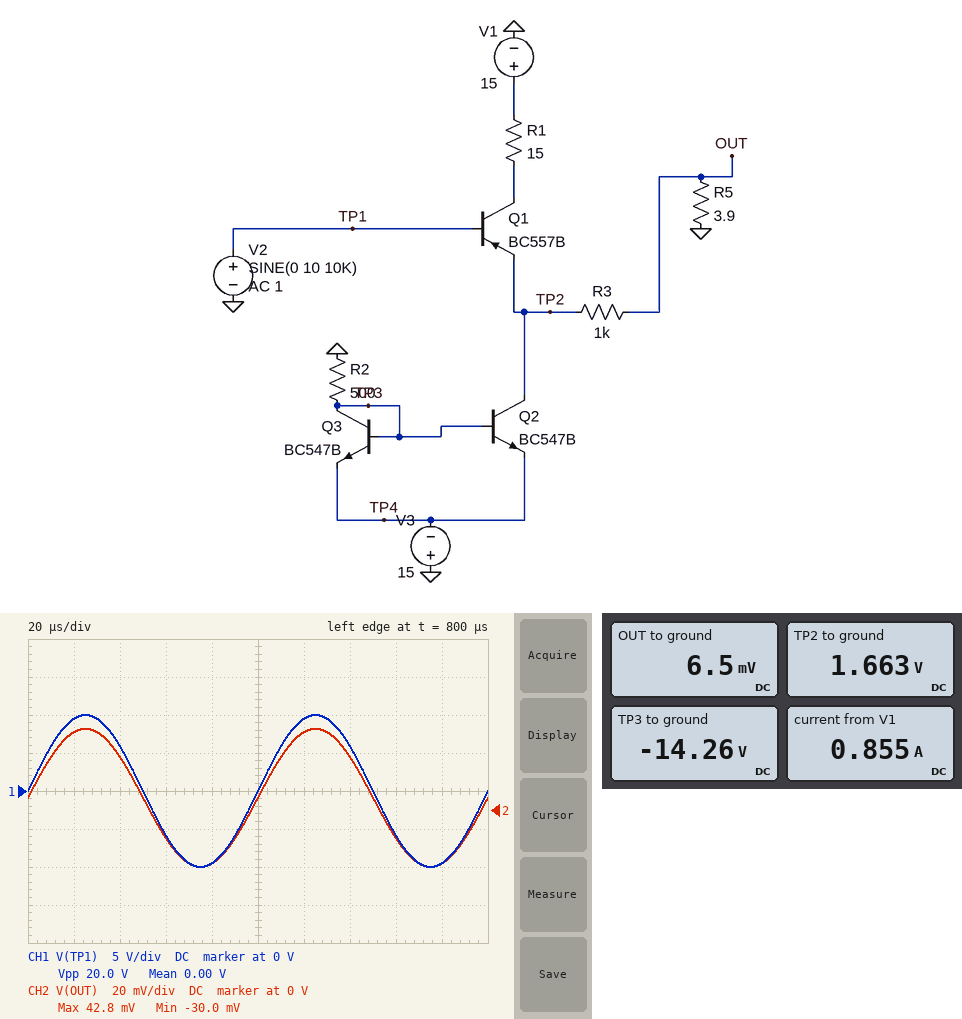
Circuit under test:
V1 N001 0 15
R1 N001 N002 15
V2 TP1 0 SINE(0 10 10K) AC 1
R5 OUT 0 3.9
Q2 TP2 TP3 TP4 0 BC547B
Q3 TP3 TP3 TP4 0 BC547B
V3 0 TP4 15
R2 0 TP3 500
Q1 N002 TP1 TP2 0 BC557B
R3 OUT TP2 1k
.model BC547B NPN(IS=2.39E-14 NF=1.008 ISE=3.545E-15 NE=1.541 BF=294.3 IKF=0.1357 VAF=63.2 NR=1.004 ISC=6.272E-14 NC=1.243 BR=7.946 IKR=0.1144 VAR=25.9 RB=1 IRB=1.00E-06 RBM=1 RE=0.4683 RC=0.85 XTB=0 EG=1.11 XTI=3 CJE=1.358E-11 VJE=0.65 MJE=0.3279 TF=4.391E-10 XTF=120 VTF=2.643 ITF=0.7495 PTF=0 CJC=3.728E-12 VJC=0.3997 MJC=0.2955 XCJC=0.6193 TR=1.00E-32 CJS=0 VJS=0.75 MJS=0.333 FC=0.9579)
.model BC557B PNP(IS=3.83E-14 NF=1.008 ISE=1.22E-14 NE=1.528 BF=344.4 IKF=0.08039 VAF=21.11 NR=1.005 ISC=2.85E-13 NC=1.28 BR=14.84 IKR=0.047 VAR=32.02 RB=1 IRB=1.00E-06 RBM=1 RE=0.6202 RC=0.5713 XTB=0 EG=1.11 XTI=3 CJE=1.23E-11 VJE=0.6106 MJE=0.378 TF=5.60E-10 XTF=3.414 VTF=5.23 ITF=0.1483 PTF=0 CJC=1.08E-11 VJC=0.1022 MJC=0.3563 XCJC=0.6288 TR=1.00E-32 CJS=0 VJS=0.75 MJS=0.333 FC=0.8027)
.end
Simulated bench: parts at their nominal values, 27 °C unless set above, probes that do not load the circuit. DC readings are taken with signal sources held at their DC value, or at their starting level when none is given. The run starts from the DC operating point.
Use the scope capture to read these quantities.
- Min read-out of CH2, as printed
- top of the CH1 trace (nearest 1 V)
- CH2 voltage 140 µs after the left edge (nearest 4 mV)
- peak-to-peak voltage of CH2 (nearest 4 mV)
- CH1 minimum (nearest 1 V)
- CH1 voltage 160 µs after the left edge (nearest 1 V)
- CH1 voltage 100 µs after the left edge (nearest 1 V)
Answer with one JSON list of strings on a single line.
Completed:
["-30.0 mV", "10 V", "28 mV", "72 mV", "-10 V", "-6 V", "0 V"]
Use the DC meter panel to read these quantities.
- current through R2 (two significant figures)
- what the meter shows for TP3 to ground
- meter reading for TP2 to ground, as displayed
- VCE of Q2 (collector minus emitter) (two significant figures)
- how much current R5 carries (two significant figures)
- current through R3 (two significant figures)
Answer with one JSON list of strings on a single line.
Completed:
["29 mA", "-14.26 V", "1.663 V", "17 V", "1.7 mA", "1.7 mA"]
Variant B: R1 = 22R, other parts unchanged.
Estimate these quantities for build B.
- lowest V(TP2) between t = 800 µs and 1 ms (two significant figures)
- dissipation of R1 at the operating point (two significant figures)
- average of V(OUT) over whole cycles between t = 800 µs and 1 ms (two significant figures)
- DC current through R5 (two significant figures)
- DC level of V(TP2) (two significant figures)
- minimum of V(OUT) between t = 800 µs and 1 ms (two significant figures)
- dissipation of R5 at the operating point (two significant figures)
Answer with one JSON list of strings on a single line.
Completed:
["-8.1 V", "8.0 W", "5.4 mV", "1.4 mA", "1.4 V", "-32 mV", "7.6 µW"]
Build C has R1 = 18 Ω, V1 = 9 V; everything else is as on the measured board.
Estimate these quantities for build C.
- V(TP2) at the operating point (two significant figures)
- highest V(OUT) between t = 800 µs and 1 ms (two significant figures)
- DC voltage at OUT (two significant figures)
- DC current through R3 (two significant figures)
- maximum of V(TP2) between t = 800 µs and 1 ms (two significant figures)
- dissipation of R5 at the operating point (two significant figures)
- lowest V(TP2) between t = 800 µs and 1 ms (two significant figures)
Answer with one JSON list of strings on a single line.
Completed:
["1.2 V", "31 mV", "4.7 mV", "1.2 mA", "8.0 V", "5.6 µW", "-15 V"]
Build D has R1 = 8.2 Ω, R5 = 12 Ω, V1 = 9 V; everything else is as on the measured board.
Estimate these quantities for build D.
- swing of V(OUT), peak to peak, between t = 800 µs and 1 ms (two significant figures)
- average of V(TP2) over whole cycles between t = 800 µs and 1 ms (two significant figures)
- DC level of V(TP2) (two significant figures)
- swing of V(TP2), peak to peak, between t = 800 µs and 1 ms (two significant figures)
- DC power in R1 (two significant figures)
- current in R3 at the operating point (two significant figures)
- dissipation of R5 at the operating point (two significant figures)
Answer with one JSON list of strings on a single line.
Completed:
["280 mV", "-3.5 V", "1.6 V", "23 V", "5.7 W", "1.6 mA", "32 µW"]
